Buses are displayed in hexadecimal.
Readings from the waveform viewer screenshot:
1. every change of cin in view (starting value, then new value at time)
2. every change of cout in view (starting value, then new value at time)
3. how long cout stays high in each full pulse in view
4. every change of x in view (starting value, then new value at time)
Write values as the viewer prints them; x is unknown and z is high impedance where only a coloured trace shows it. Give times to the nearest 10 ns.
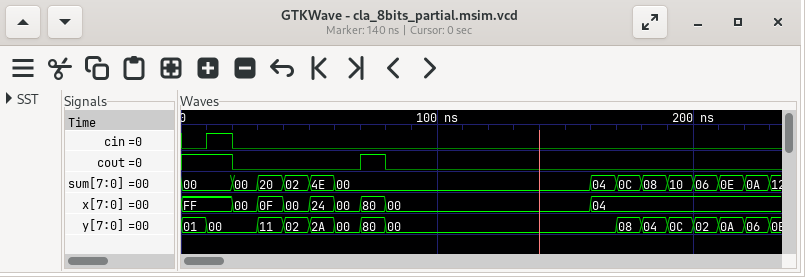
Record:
0, 1 at 10 ns, 0 at 20 ns
1, 0 at 20 ns, 1 at 70 ns, 0 at 80 ns
10 ns
FF, 00 at 20 ns, 0F at 30 ns, 00 at 40 ns, 24 at 50 ns, 00 at 60 ns, 80 at 70 ns, 00 at 80 ns, 04 at 160 ns
